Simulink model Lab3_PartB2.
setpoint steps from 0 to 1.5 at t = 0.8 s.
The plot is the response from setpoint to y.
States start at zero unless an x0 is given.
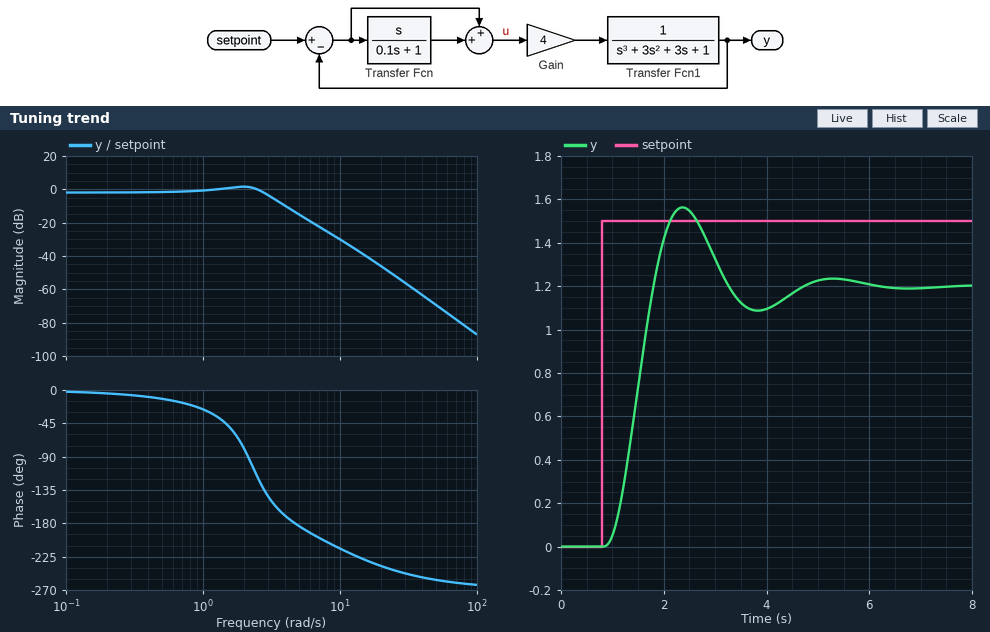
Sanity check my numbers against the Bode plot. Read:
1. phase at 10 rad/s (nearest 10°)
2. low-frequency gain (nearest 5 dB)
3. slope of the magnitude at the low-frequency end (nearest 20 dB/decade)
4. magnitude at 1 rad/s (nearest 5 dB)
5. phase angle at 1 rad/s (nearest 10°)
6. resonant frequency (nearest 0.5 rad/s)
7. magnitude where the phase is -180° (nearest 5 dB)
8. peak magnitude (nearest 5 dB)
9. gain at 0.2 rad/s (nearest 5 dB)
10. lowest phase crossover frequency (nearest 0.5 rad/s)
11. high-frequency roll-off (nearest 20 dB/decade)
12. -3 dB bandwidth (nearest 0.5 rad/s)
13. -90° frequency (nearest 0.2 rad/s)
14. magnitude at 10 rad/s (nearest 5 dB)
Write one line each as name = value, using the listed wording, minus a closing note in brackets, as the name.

phase at 10 rad/s = -210°
low-frequency gain = 0 dB
slope of the magnitude at the low-frequency end = 0 dB/decade
magnitude at 1 rad/s = 0 dB
phase angle at 1 rad/s = -30°
resonant frequency = 2.0 rad/s
magnitude where the phase is -180° = -15 dB
peak magnitude = 0 dB
gain at 0.2 rad/s = 0 dB
lowest phase crossover frequency = 4.5 rad/s
high-frequency roll-off = -60 dB/decade
-3 dB bandwidth = 3.0 rad/s
-90° frequency = 2.2 rad/s
magnitude at 10 rad/s = -30 dB
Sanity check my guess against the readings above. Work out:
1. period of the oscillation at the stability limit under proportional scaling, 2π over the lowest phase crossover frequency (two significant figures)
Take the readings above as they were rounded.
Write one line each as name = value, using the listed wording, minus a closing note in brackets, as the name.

period of the oscillation at the stability limit under proportional scaling, 2π over the lowest phase crossover frequency = 1.4 s
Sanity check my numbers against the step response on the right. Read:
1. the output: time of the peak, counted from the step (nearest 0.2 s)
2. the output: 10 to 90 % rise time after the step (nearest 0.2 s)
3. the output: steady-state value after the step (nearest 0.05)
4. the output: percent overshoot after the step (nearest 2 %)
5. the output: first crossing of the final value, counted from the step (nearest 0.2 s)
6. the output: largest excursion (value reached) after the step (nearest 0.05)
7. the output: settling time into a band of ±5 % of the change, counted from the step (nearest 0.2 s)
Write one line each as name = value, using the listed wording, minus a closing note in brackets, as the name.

the output: time of the peak, counted from the step = 1.6 s
the output: 10 to 90 % rise time after the step = 0.6 s
the output: steady-state value after the step = 1.20
the output: percent overshoot after the step = 30 %
the output: first crossing of the final value, counted from the step = 1.0 s
the output: largest excursion (value reached) after the step = 1.55
the output: settling time into a band of ±5 % of the change, counted from the step = 3.6 s
